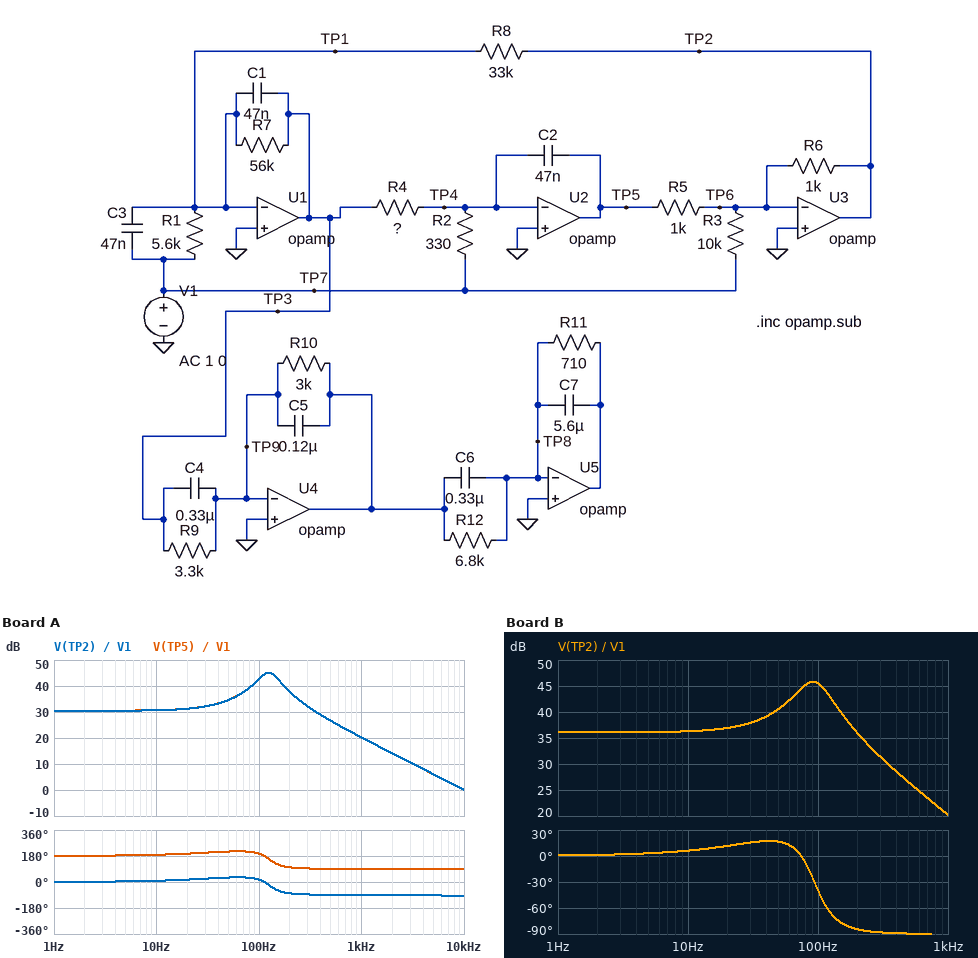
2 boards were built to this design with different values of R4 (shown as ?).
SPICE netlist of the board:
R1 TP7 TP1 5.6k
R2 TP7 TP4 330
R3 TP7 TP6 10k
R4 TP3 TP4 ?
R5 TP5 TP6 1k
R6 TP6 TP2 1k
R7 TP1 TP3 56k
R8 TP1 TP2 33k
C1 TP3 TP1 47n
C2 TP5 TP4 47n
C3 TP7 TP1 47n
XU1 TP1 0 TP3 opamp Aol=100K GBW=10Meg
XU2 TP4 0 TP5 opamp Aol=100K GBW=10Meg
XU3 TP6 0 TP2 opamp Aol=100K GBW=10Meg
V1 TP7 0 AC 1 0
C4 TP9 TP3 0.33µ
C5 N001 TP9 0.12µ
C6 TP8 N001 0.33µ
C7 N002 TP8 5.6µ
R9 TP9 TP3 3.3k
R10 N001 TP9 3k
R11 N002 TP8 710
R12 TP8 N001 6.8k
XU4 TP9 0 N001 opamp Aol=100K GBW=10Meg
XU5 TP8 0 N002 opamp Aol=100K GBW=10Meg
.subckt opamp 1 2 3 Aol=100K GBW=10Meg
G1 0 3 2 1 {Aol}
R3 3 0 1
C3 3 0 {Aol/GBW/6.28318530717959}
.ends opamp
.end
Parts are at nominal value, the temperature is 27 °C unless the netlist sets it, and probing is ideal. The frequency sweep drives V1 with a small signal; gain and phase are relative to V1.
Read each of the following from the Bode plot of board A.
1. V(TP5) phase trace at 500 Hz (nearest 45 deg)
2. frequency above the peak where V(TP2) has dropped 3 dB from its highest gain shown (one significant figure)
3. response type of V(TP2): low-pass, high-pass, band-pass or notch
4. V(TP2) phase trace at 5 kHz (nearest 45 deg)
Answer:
90 deg
200 Hz
band-pass
-90 deg
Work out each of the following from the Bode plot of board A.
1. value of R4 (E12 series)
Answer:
22 kΩ
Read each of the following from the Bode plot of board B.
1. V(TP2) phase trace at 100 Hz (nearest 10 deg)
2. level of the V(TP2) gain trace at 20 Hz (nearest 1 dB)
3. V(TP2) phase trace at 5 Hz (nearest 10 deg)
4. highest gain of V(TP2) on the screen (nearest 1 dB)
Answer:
-40 deg
37 dB
0 deg
46 dB
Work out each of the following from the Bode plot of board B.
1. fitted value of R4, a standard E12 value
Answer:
39 kΩ
